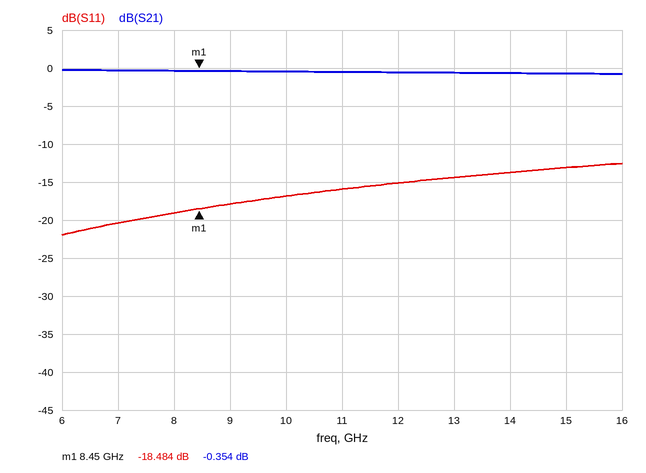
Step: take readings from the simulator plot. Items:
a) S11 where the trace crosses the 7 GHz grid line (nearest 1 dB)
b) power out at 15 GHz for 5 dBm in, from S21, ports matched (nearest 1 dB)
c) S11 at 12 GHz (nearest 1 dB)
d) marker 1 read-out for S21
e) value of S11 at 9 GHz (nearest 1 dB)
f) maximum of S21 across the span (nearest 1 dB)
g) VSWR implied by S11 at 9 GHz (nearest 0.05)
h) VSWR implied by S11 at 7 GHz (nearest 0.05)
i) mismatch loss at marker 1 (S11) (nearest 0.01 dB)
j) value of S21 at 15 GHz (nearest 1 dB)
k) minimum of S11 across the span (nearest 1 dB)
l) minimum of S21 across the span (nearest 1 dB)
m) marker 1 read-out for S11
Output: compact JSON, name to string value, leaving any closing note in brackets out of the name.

{"S11 where the trace crosses the 7 GHz grid line": "-20 dB", "power out at 15 GHz for 5 dBm in, from S21, ports matched": "4 dBm", "S11 at 12 GHz": "-15 dB", "marker 1 read-out for S21": "-0.354 dB", "value of S11 at 9 GHz": "-18 dB", "maximum of S21 across the span": "0 dB", "VSWR implied by S11 at 9 GHz": "1.30", "VSWR implied by S11 at 7 GHz": "1.20", "mismatch loss at marker 1 (S11)": "0.06 dB", "value of S21 at 15 GHz": "-1 dB", "minimum of S11 across the span": "-22 dB", "minimum of S21 across the span": "-1 dB", "marker 1 read-out for S11": "-18.484 dB"}
